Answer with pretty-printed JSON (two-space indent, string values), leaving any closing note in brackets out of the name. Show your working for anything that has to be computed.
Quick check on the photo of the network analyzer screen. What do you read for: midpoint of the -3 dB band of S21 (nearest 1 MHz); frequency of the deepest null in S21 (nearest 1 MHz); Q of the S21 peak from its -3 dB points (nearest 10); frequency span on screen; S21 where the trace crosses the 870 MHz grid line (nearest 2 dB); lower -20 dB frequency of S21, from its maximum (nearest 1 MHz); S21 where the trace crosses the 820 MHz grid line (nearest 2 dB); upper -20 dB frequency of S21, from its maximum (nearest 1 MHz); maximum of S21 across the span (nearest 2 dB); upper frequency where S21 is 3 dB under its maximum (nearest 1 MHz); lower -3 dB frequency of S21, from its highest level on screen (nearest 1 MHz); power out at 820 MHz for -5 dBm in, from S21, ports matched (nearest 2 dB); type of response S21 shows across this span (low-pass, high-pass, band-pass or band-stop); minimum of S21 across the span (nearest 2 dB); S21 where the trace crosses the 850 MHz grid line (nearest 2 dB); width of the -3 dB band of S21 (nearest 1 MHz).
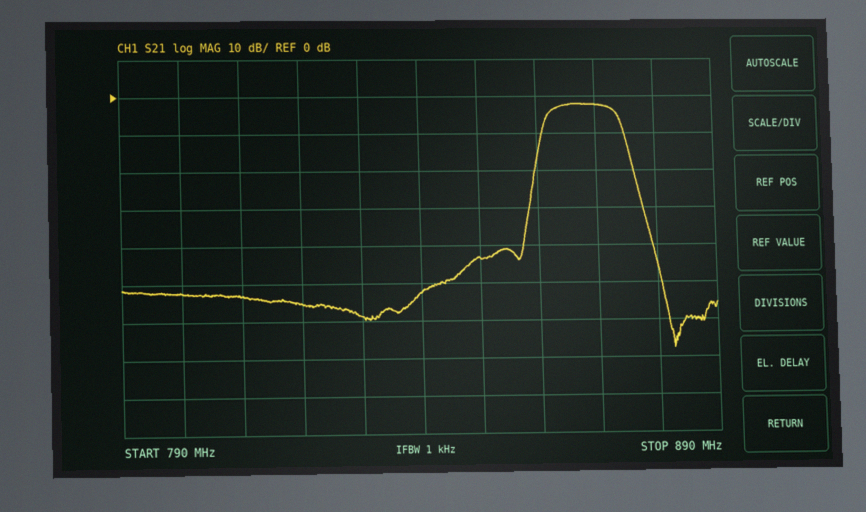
{
  "midpoint of the -3 dB band of S21": "868 MHz",
  "frequency of the deepest null in S21": "883 MHz",
  "Q of the S21 peak from its -3 dB points": "868 MHz / 12 MHz ≈ 72.3, so 70 to the nearest 10",
  "frequency span on screen": "100 MHz",
  "S21 where the trace crosses the 870 MHz grid line": "-2 dB",
  "lower -20 dB frequency of S21, from its maximum": "859 MHz",
  "S21 where the trace crosses the 820 MHz grid line": "-56 dB",
  "upper -20 dB frequency of S21, from its maximum": "877 MHz",
  "maximum of S21 across the span": "-2 dB",
  "upper frequency where S21 is 3 dB under its maximum": "874 MHz",
  "lower -3 dB frequency of S21, from its highest level on screen": "862 MHz",
  "power out at 820 MHz for -5 dBm in, from S21, ports matched": "-5 dBm + (-56 dB) = -60 dBm",
  "type of response S21 shows across this span": "band-pass",
  "minimum of S21 across the span": "-68 dB",
  "S21 where the trace crosses the 850 MHz grid line": "-44 dB",
  "width of the -3 dB band of S21": "874 MHz − 862 MHz = 12 MHz"
}
